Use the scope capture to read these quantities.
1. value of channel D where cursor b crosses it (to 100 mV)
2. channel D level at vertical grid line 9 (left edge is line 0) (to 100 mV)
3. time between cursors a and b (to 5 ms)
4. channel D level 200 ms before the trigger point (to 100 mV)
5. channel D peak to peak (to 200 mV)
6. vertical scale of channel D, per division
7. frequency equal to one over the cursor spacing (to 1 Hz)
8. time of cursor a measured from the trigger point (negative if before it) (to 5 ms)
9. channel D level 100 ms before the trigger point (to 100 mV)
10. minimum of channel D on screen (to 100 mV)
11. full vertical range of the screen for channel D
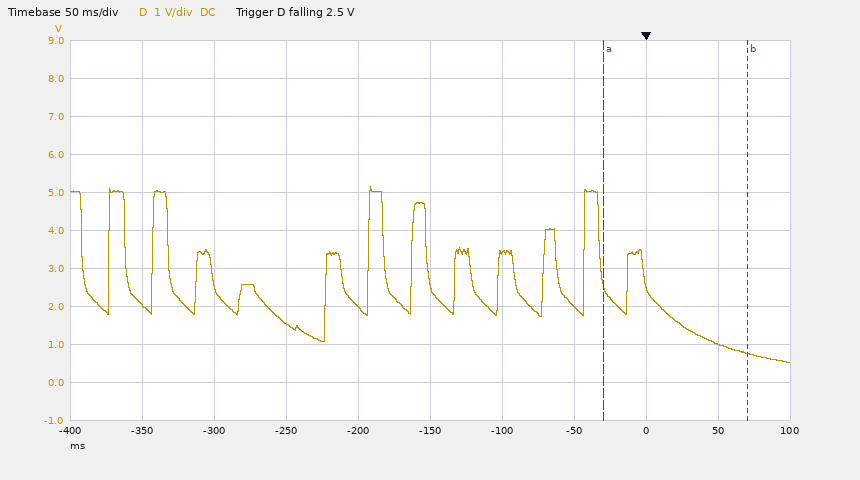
800 mV
1.0 V
100 ms
2.0 V
4.6 V
1 V
10 Hz
-30 ms
3.4 V
500 mV
10 V
